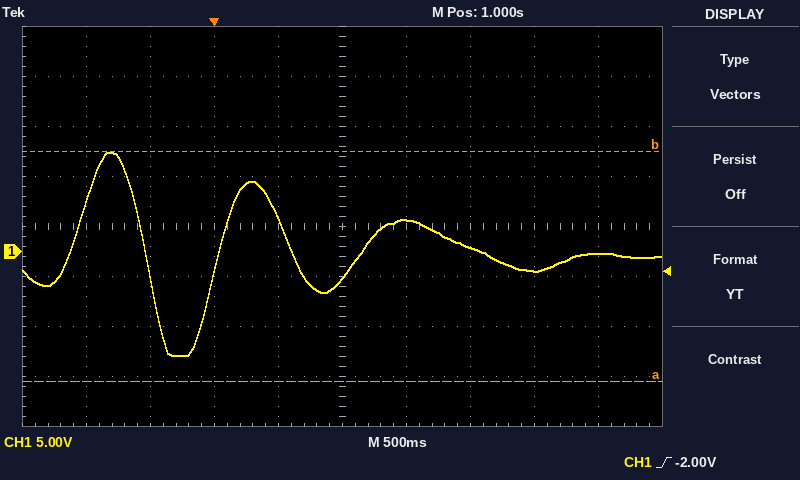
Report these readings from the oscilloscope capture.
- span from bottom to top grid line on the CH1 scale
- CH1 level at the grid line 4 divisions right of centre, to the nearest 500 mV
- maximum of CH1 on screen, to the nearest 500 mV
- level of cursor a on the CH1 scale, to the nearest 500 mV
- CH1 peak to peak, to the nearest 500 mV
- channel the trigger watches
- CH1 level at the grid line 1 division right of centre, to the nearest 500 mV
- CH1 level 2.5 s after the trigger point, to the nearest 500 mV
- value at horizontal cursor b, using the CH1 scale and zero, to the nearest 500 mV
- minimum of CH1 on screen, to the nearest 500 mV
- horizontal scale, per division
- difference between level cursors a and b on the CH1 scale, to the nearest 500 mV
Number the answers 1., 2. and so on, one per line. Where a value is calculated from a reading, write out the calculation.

1. 40 V
2. 0.0 V
3. 10.0 V
4. -13.0 V
5. 10.0 V − (-10.5 V) = 20.5 V
6. CH1
7. 3.0 V
8. -2.0 V
9. 10.0 V
10. -10.5 V
11. 500 ms
12. 23.0 V
